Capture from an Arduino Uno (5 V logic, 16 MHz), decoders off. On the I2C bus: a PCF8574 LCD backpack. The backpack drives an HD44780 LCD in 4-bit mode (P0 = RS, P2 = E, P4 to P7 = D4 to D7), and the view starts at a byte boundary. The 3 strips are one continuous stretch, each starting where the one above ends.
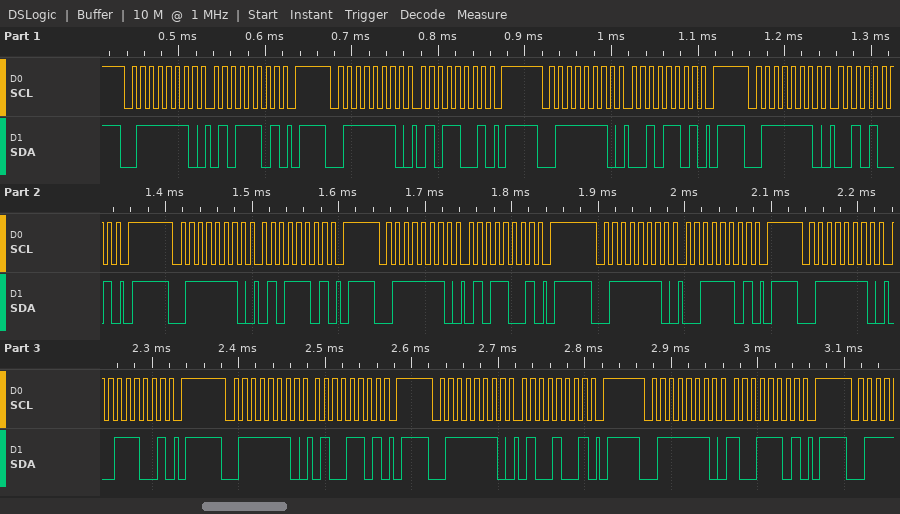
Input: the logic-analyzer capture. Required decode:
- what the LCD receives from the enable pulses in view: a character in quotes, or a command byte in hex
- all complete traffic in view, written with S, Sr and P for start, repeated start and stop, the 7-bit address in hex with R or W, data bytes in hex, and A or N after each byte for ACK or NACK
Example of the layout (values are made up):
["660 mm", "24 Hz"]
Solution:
["'R' 'S'", "S 3FW A 5D A P S 3FW A 59 A P S 3FW A 2D A P S 3FW A 29 A P S 3FW A 5D A P S 3FW A 59 A P S 3FW A 3D A P S 3FW A 39 A P S 3FW A 4D A P S 3FW A 49 A P S 3FW A 9D A P"]
